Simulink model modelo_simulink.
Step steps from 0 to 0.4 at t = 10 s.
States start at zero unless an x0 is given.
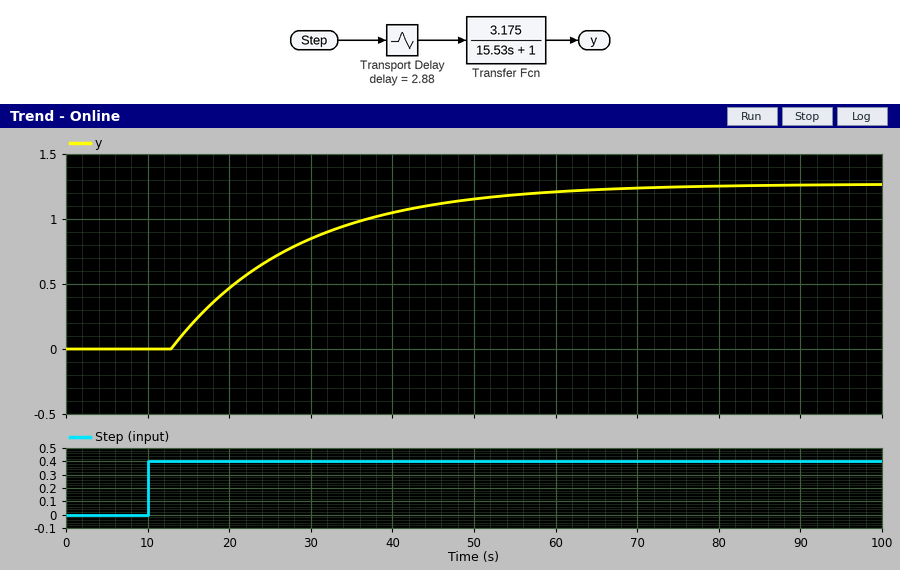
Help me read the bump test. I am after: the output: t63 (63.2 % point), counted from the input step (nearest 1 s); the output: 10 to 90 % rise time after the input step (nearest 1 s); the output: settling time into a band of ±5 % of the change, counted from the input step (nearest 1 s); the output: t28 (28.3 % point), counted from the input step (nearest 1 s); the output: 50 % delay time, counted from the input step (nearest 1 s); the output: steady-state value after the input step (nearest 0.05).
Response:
18 s
34 s
49 s
8 s
14 s
1.25
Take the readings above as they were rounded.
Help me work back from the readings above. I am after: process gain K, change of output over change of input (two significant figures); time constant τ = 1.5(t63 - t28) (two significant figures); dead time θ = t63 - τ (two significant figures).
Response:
3.1
15 s
3.0 s
